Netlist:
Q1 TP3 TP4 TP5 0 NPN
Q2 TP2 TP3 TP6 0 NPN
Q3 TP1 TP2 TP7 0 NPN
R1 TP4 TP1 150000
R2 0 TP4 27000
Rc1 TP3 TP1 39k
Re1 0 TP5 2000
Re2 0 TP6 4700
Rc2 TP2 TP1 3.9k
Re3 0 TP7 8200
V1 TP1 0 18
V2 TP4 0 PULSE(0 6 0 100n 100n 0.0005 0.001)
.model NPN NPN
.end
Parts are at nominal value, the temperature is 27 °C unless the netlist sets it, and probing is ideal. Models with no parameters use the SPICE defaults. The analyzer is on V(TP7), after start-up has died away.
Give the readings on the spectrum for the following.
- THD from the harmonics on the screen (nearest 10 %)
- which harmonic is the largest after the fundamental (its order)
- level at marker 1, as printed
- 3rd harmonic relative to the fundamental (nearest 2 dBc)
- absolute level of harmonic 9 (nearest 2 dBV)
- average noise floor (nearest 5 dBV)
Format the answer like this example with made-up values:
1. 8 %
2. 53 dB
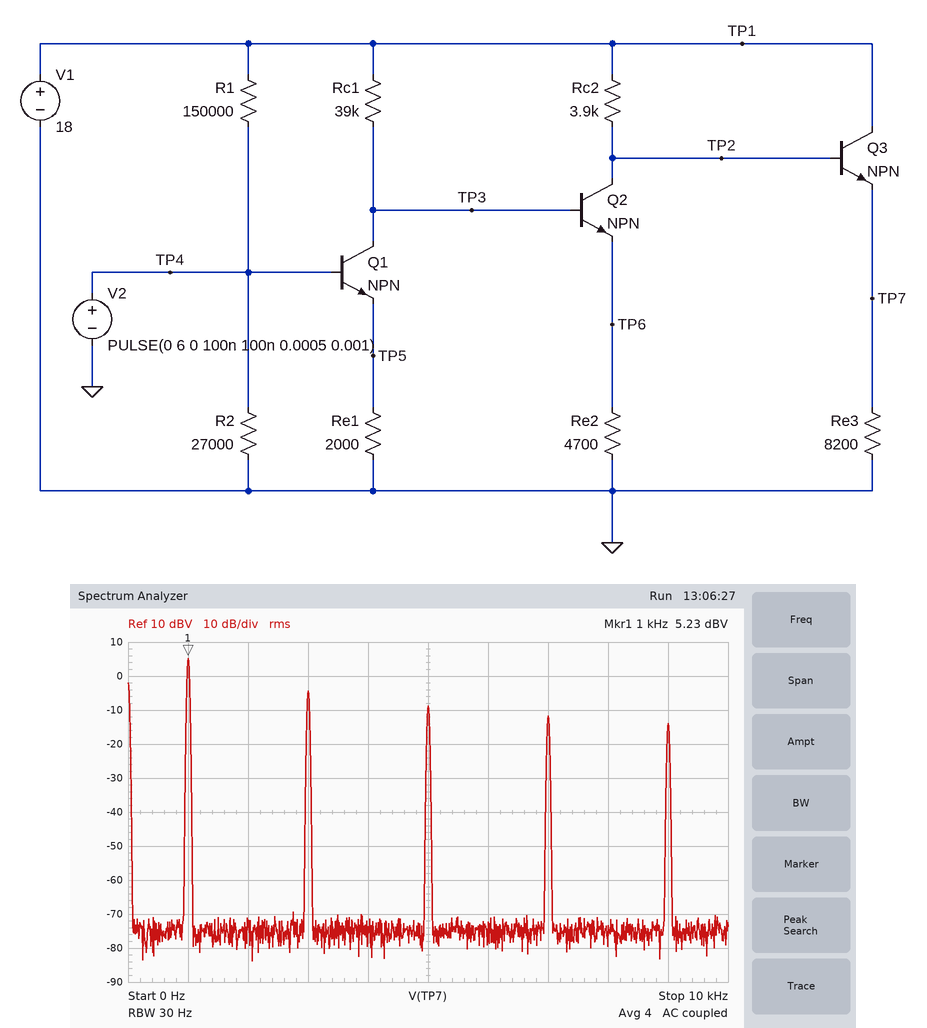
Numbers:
1. 40 %
2. 3
3. 5.23 dBV
4. -10 dBc
5. -14 dBV
6. -75 dBV
